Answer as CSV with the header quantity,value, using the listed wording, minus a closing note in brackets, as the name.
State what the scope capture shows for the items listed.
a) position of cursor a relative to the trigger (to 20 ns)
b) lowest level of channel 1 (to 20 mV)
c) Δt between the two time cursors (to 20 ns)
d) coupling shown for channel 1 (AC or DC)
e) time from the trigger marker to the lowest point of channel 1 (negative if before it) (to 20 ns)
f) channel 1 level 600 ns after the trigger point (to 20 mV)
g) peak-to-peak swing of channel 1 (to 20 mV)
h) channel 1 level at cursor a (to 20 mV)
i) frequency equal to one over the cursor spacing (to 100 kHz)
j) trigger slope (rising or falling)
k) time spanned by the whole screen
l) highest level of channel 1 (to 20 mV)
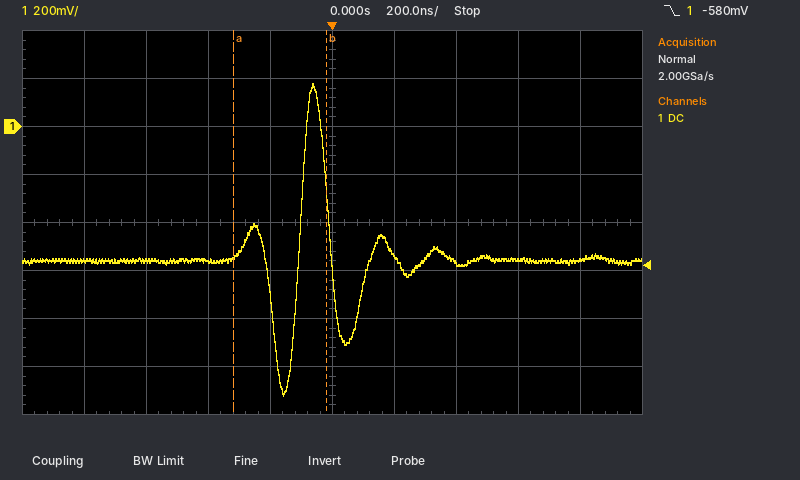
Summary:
quantity,value
position of cursor a relative to the trigger,-320 ns
lowest level of channel 1,-1.12 V
Δt between the two time cursors,300 ns
coupling shown for channel 1,DC
time from the trigger marker to the lowest point of channel 1 (negative if before it),-160 ns
channel 1 level 600 ns after the trigger point,-560 mV
peak-to-peak swing of channel 1,1.30 V
channel 1 level at cursor a,-540 mV
frequency equal to one over the cursor spacing,3.3 MHz
trigger slope,falling
time spanned by the whole screen,2 µs
highest level of channel 1,180 mV
